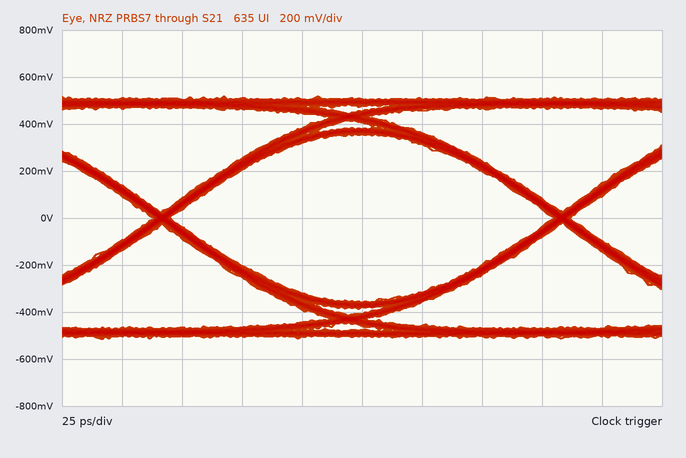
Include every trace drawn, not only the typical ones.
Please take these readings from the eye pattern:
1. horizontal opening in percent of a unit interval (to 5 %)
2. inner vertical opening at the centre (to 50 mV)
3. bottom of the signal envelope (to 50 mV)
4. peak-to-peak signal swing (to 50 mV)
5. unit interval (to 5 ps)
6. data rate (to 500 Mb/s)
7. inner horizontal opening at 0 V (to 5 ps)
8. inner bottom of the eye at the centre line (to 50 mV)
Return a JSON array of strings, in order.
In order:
["95 %", "700 mV", "-500 mV", "1.05 V", "165 ps", "6.0 Gb/s", "160 ps", "-350 mV"]
